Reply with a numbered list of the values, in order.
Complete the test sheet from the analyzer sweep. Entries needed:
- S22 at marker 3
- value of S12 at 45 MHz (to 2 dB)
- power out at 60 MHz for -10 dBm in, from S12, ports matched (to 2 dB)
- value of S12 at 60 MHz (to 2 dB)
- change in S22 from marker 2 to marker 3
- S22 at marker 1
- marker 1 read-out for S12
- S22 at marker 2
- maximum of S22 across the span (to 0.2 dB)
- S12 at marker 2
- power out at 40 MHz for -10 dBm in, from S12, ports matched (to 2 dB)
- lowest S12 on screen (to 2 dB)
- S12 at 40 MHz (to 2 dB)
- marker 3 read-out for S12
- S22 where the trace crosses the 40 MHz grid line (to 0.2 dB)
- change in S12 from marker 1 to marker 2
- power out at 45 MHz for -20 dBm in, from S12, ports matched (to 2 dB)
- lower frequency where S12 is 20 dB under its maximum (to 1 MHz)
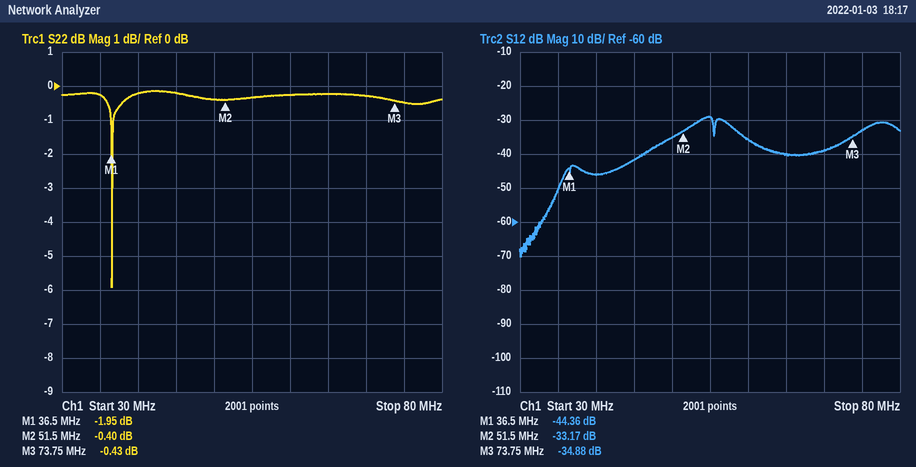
1. -0.43 dB
2. -42 dB
3. -46 dBm
4. -36 dB
5. -0.03 dB
6. -1.95 dB
7. -44.36 dB
8. -0.40 dB
9. -0.2 dB
10. -33.17 dB
11. -56 dBm
12. -70 dB
13. -46 dB
14. -34.88 dB
15. -0.2 dB
16. 11.19 dB
17. -62 dBm
18. 35 MHz
